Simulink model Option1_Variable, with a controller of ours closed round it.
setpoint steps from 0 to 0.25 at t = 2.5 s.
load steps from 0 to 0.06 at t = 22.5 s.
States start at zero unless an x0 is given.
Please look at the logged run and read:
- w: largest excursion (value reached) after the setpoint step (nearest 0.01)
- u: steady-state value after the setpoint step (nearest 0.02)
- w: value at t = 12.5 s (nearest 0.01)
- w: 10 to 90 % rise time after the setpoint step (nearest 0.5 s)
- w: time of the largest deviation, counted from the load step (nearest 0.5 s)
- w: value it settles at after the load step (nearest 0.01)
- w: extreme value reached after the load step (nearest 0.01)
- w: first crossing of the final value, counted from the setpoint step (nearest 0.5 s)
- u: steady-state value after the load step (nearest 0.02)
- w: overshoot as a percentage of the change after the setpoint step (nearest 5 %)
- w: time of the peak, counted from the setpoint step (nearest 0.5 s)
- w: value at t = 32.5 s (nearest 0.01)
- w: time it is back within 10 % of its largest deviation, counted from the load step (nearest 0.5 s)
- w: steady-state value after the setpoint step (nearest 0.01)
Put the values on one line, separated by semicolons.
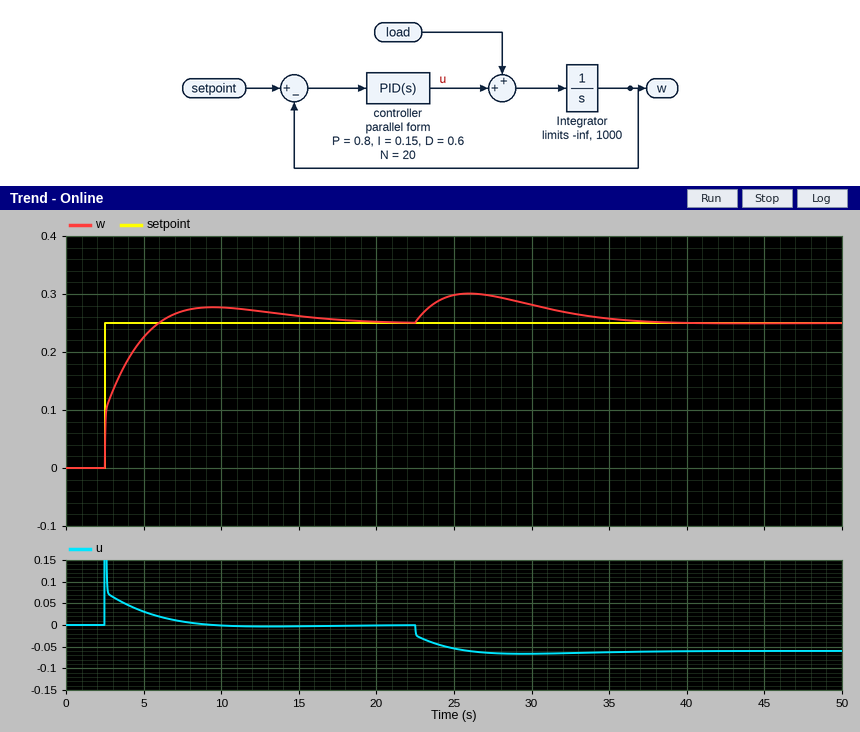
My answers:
0.28; 0.00; 0.27; 2.5 s; 3.5 s; 0.25; 0.30; 3.5 s; -0.06; 10 %; 7.0 s; 0.27; 13.5 s; 0.25
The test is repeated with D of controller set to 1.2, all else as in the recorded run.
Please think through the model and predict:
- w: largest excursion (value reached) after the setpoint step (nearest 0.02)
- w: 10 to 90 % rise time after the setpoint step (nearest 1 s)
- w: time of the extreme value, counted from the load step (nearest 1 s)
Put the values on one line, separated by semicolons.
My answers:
0.28; 3 s; 4 s
